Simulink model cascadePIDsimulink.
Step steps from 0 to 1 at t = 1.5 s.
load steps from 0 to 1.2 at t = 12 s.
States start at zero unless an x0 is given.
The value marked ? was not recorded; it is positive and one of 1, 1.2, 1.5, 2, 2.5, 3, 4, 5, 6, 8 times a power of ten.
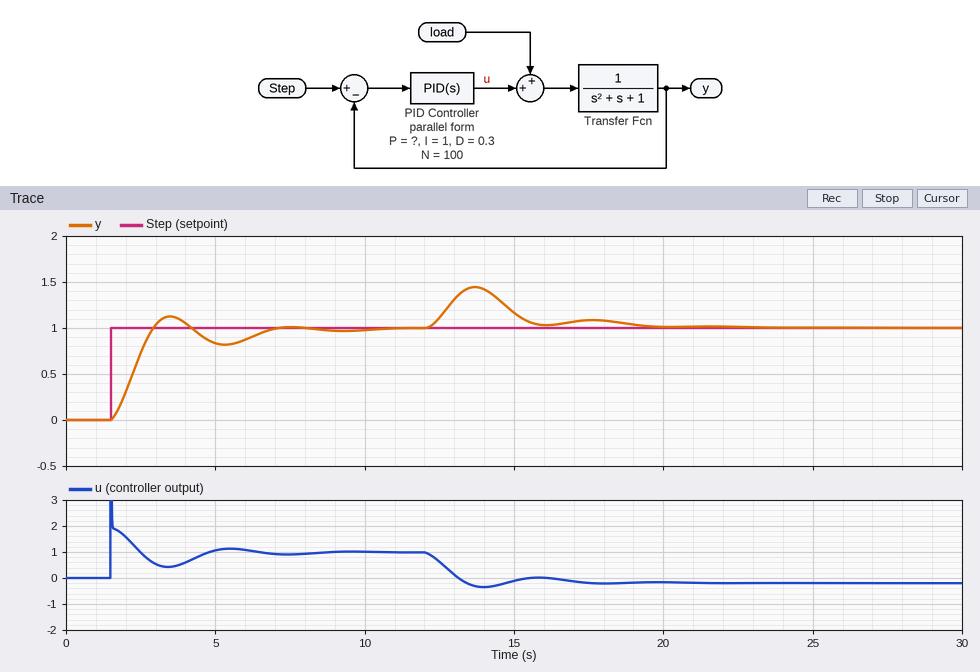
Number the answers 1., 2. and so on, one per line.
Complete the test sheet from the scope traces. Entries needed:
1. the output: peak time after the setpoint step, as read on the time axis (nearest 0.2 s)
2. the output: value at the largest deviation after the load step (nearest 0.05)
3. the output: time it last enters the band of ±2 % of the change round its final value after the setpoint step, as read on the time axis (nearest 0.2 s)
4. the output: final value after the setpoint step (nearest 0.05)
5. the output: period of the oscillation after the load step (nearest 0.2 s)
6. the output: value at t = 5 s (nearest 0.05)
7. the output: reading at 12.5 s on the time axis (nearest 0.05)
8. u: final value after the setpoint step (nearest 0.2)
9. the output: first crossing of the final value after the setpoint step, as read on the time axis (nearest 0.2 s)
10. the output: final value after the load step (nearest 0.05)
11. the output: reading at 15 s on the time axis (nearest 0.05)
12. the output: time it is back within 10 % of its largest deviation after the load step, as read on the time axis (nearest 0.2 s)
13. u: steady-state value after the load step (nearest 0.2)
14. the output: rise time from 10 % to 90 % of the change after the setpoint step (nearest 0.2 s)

1. 3.4 s
2. 1.45
3. 10.2 s
4. 1.00
5. 4.0 s
6. 0.85
7. 1.10
8. 1.0
9. 3.0 s
10. 1.00
11. 1.15
12. 18.8 s
13. -0.2
14. 1.0 s
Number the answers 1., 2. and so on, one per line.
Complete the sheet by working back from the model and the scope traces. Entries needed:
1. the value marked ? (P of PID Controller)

1. 2
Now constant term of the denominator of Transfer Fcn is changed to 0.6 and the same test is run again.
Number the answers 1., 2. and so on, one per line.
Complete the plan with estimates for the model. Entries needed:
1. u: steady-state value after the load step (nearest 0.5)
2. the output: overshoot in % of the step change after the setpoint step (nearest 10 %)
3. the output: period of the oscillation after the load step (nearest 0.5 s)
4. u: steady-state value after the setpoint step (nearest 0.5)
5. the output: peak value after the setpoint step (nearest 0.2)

1. -0.5
2. 30 %
3. 4.5 s
4. 0.5
5. 1.2
